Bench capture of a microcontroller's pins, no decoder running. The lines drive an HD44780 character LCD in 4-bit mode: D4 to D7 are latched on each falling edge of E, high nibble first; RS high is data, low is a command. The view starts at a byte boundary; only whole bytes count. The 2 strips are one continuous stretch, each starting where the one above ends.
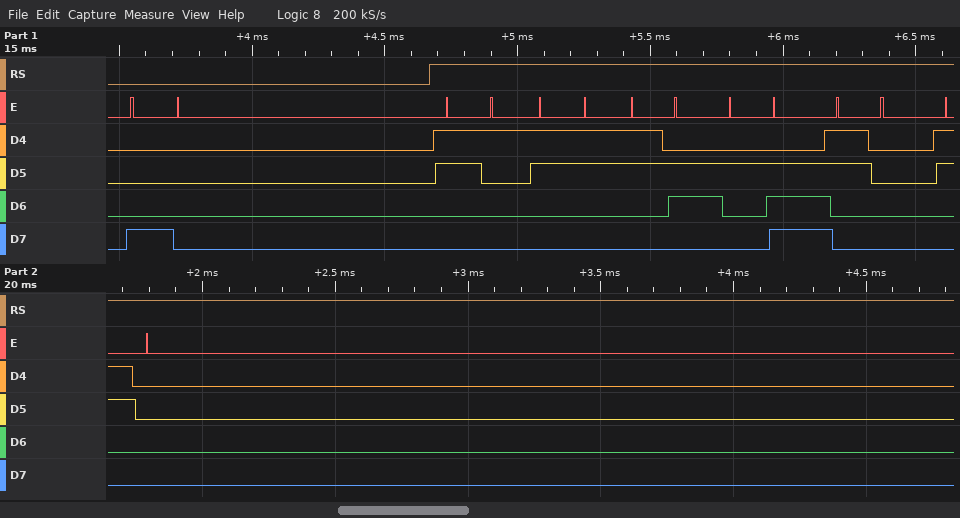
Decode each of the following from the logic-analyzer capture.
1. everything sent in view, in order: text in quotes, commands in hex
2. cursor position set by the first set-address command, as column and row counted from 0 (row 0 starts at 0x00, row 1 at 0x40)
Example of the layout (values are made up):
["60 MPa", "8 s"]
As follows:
["0x80 \"136.00\"", "column 0, row 0"]
